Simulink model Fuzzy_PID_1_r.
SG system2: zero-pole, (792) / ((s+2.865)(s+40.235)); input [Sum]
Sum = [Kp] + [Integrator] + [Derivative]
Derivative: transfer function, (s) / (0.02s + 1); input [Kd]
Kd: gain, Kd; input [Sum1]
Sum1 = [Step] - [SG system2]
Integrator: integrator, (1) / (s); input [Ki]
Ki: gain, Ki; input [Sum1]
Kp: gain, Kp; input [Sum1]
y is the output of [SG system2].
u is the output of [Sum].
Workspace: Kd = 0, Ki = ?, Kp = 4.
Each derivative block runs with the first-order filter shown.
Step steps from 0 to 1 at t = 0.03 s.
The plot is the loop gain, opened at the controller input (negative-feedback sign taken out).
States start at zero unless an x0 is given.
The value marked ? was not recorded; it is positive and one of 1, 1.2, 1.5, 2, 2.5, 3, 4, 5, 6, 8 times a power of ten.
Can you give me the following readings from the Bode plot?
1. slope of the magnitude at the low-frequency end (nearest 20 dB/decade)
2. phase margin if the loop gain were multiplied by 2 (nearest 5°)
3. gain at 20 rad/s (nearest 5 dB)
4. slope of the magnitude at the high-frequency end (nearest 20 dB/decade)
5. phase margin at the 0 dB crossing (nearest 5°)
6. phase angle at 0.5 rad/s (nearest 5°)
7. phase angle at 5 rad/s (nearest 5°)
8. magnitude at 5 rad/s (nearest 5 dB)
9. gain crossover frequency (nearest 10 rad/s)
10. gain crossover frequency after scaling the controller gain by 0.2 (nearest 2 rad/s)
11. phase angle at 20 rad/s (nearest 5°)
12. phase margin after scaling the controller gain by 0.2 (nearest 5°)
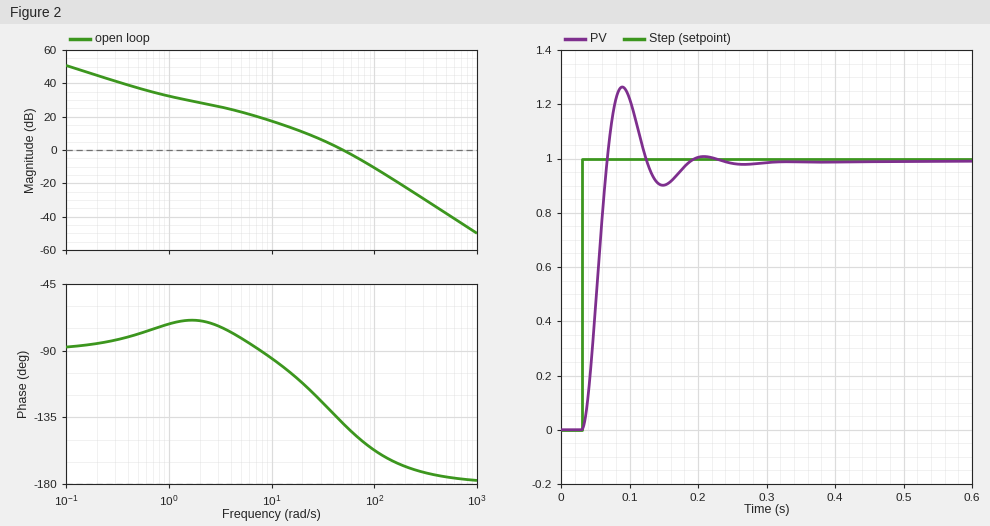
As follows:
-20 dB/decade
30°
10 dB
-40 dB/decade
40°
-80°
-80°
25 dB
50 rad/s
14 rad/s
-110°
75°
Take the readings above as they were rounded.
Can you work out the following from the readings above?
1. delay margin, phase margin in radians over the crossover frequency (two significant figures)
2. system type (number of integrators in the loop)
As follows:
0.014 s
1
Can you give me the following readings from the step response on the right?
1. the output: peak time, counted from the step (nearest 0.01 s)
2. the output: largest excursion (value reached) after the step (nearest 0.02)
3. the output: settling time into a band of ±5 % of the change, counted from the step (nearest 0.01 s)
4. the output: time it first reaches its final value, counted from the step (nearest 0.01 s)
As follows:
0.06 s
1.26
0.14 s
0.04 s
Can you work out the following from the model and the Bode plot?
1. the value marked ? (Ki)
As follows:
5
